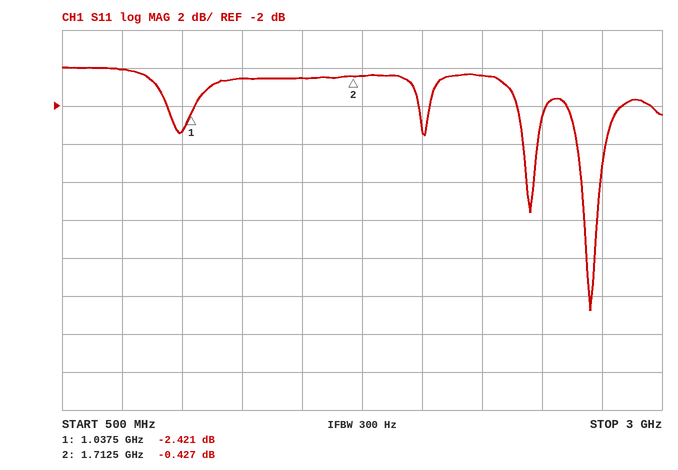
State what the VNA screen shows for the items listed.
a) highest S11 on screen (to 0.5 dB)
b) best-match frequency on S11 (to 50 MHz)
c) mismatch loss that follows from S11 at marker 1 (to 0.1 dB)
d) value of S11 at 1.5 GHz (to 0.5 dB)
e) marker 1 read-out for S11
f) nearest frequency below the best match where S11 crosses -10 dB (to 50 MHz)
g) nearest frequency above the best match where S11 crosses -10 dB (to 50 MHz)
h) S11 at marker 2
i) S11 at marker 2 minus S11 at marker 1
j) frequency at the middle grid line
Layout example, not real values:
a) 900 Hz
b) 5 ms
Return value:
a) 0.0 dB
b) 2.70 GHz
c) 3.7 dB
d) -0.5 dB
e) -2.421 dB
f) 2.70 GHz
g) 2.70 GHz
h) -0.427 dB
i) 1.994 dB
j) 1.75 GHz
